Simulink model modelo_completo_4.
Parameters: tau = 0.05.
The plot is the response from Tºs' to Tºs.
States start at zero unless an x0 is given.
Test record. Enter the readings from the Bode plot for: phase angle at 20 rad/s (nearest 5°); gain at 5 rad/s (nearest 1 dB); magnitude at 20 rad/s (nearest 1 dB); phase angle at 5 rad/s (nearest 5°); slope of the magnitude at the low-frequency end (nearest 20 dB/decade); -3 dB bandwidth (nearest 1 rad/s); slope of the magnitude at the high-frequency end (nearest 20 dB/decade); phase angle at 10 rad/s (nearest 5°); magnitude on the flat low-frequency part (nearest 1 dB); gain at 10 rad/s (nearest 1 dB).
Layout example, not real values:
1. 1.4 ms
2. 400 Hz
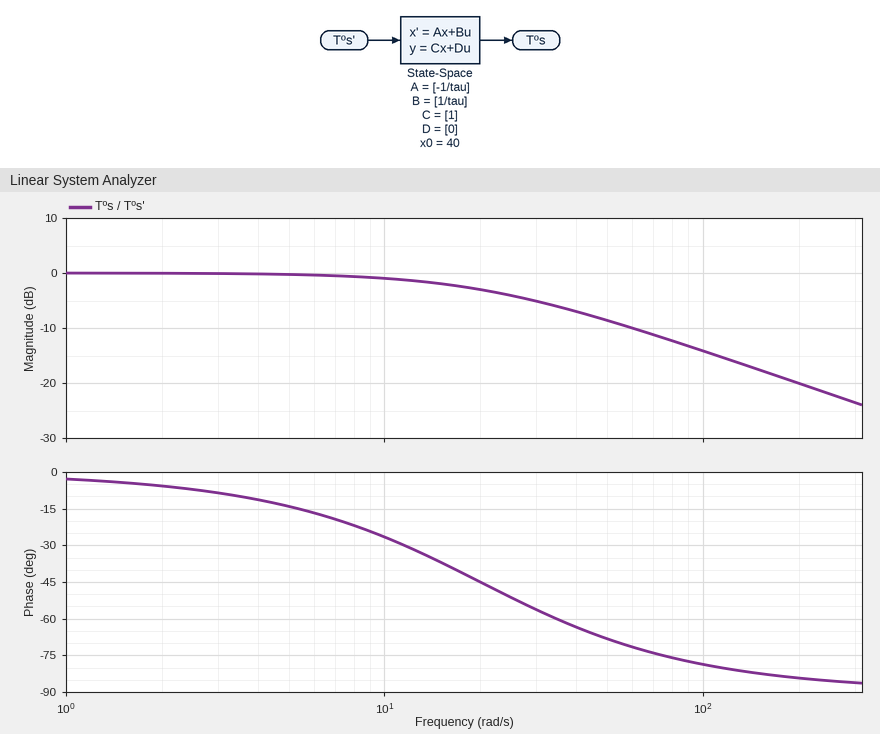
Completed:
1. -45°
2. 0 dB
3. -3 dB
4. -15°
5. 0 dB/decade
6. 20 rad/s
7. -20 dB/decade
8. -25°
9. 0 dB
10. -1 dB
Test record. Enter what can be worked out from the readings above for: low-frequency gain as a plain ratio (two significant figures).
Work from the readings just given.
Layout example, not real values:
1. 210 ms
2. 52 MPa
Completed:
1. 1.0
